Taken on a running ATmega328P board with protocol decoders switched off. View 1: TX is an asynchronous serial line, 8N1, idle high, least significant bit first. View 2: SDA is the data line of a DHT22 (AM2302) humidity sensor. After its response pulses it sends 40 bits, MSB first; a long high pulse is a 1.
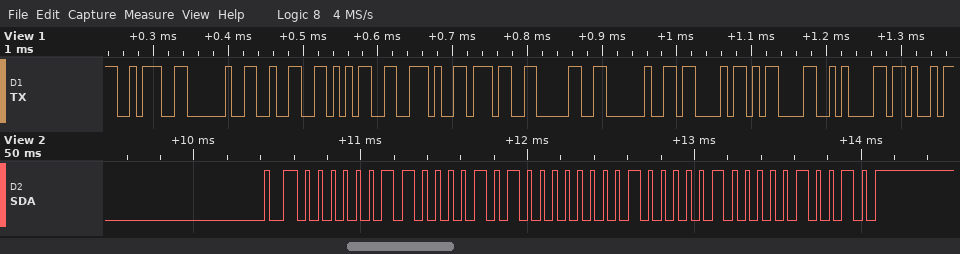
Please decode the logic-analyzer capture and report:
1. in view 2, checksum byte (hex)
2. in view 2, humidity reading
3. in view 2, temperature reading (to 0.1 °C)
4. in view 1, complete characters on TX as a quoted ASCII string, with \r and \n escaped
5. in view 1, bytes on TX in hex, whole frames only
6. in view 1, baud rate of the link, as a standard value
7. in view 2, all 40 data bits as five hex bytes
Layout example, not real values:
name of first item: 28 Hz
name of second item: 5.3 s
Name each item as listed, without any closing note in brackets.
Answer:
in view 2, checksum byte: 0x12
in view 2, humidity reading: 77.8 %
in view 2, temperature reading: 26.0 °C
in view 1, complete characters on TX as a quoted ASCII string, with \r and \n escaped: ": 25.70 C\r\nK"
in view 1, bytes on TX in hex, whole frames only: 3A 20 32 35 2E 37 30 20 43 0D 0A 4B
in view 1, baud rate of the link, as a standard value: 115200 baud
in view 2, all 40 data bits as five hex bytes: 03 0A 01 04 12
